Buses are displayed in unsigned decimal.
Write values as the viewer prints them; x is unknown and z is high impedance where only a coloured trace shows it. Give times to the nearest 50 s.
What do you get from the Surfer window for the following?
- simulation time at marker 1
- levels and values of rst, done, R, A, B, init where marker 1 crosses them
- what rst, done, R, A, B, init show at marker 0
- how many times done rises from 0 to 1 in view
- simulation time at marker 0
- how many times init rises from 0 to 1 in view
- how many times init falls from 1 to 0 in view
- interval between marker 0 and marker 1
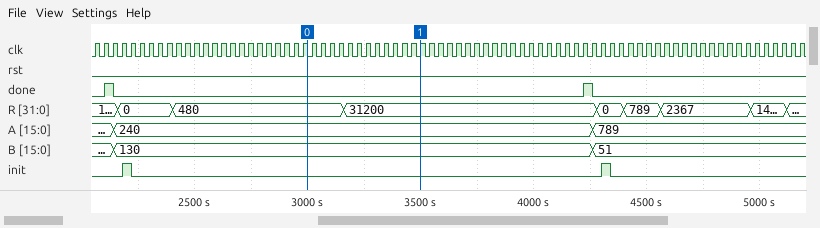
3500 s
rst=0, done=0, R=31200, A=240, B=130, init=0
rst=0, done=0, R=480, A=240, B=130, init=0
2
3000 s
2
2
500 s
